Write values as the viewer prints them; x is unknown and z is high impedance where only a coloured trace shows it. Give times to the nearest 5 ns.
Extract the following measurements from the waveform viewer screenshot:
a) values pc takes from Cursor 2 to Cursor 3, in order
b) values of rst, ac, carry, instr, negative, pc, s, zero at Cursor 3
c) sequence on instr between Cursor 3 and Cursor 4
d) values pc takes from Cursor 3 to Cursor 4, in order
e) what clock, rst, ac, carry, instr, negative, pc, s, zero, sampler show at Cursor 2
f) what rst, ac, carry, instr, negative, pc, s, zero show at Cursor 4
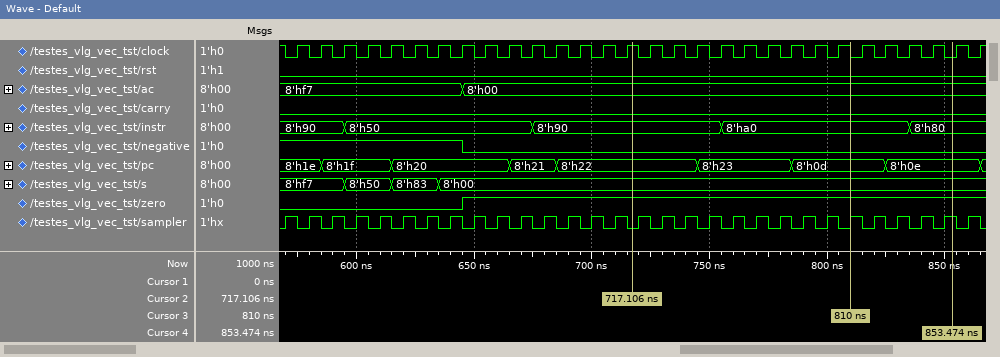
8'h22, 8'h23, 8'h0d
rst=0, ac=8'h00, carry=0, instr=8'ha0, negative=0, pc=8'h0d, s=8'h00, zero=1
8'ha0, 8'h80
8'h0d, 8'h0e
clock=1, rst=0, ac=8'h00, carry=0, instr=8'h90, negative=0, pc=8'h22, s=8'h00, zero=1, sampler=0
rst=0, ac=8'h00, carry=0, instr=8'h80, negative=0, pc=8'h0e, s=8'h00, zero=1
